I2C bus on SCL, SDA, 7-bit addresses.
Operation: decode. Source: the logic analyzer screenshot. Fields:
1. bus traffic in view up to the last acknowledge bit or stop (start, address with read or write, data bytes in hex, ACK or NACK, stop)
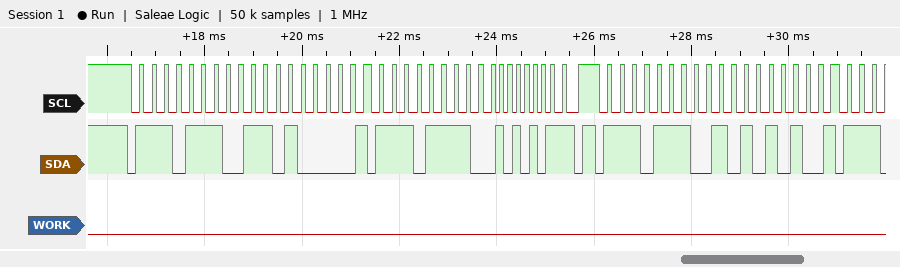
start, address 77 write ACK, D0 ACK, repeated start, address 77 read ACK, 55 NACK, stop, start, address 77 write ACK, AA ACK
